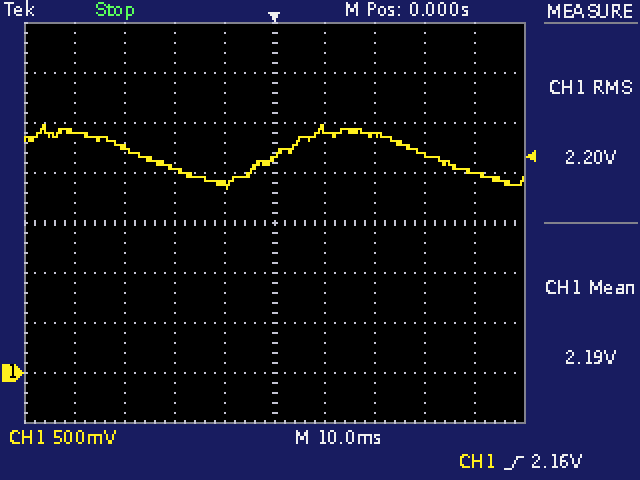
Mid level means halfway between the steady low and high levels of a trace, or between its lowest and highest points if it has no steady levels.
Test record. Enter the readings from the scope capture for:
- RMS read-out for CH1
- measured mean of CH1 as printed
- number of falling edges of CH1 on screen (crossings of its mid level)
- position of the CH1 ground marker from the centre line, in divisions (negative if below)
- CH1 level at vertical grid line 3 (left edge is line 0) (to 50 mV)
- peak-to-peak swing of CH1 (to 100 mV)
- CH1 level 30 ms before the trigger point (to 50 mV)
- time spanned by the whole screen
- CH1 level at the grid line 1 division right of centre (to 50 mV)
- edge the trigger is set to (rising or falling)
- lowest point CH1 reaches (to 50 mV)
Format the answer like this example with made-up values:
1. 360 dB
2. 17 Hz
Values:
1. 2.20 V
2. 2.19 V
3. 2
4. -3.0 div
5. 2.05 V
6. 600 mV
7. 2.25 V
8. 100 ms
9. 2.45 V
10. rising
11. 1.85 V
